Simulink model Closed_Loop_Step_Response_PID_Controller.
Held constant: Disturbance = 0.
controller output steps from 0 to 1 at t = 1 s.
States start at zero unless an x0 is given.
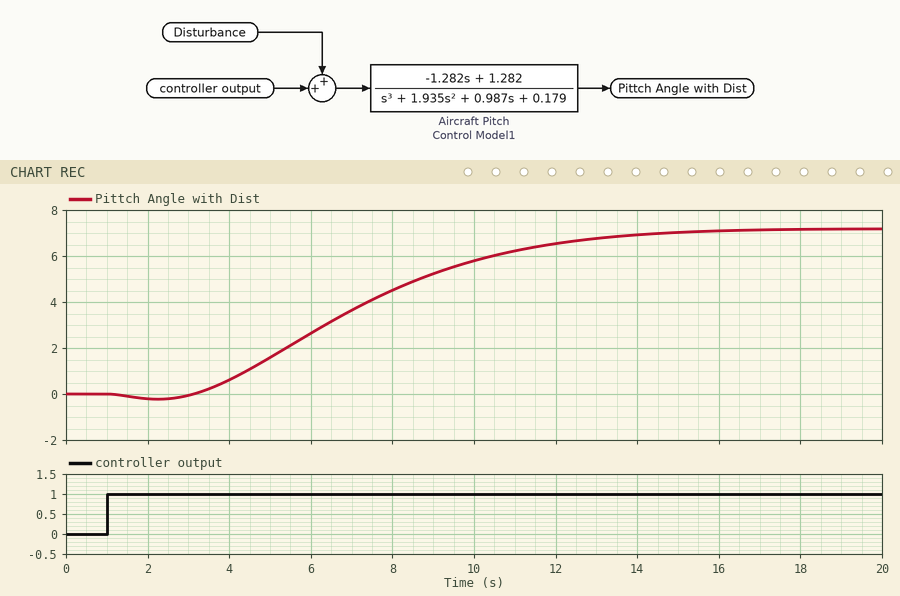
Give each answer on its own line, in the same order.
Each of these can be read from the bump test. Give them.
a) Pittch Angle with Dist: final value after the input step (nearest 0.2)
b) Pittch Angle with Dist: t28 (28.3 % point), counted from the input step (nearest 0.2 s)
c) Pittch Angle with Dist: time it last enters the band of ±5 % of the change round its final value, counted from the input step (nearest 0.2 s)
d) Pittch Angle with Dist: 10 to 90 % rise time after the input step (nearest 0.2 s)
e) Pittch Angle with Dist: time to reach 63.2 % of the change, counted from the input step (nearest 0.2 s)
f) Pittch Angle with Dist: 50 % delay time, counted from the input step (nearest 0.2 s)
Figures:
7.2
4.4 s
12.2 s
7.6 s
7.0 s
6.0 s
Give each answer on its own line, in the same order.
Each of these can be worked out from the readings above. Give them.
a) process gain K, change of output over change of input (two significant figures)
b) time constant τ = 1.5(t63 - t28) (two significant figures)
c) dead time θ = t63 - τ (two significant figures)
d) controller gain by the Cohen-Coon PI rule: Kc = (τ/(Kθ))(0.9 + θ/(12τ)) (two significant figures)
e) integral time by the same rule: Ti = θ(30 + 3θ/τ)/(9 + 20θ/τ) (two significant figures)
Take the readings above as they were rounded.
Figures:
7.2
3.9 s
3.1 s
0.17
4.0 s
